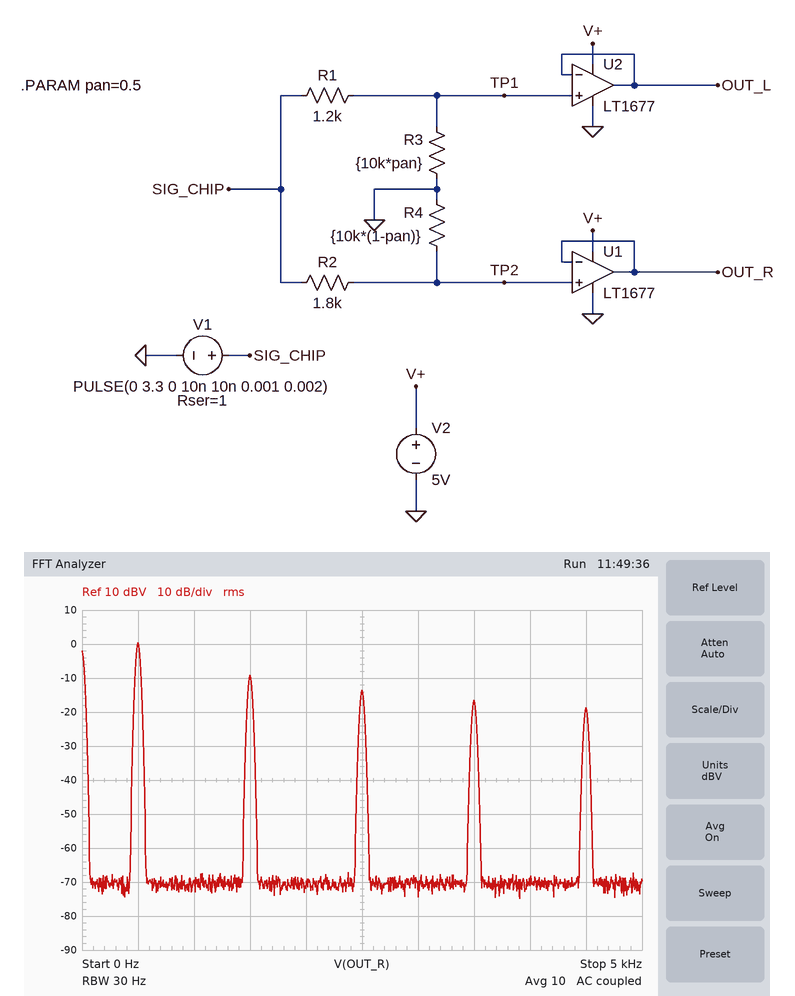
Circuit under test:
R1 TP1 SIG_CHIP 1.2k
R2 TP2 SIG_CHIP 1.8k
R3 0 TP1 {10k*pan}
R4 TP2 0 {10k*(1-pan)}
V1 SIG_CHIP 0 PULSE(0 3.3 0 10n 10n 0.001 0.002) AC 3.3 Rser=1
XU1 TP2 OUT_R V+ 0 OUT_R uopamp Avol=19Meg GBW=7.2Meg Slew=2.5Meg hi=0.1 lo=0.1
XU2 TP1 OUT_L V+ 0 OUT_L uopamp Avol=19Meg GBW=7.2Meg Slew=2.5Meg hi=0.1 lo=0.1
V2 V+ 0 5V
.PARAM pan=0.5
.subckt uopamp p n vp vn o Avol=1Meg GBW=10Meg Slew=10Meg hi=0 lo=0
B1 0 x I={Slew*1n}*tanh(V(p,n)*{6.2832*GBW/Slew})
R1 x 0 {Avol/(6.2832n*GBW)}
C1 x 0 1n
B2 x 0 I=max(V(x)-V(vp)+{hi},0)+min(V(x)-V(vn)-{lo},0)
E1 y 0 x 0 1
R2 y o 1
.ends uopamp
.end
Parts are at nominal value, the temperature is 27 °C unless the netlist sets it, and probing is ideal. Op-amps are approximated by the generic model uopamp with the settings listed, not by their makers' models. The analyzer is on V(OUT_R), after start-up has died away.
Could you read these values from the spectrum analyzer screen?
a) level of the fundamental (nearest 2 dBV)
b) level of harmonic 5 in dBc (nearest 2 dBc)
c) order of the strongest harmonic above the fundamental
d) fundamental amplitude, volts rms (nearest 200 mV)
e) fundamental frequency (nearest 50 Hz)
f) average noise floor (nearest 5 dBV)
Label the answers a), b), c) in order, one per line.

a) 0 dBV
b) -14 dBc
c) 3
d) 1.0 V
e) 500 Hz
f) -70 dBV
